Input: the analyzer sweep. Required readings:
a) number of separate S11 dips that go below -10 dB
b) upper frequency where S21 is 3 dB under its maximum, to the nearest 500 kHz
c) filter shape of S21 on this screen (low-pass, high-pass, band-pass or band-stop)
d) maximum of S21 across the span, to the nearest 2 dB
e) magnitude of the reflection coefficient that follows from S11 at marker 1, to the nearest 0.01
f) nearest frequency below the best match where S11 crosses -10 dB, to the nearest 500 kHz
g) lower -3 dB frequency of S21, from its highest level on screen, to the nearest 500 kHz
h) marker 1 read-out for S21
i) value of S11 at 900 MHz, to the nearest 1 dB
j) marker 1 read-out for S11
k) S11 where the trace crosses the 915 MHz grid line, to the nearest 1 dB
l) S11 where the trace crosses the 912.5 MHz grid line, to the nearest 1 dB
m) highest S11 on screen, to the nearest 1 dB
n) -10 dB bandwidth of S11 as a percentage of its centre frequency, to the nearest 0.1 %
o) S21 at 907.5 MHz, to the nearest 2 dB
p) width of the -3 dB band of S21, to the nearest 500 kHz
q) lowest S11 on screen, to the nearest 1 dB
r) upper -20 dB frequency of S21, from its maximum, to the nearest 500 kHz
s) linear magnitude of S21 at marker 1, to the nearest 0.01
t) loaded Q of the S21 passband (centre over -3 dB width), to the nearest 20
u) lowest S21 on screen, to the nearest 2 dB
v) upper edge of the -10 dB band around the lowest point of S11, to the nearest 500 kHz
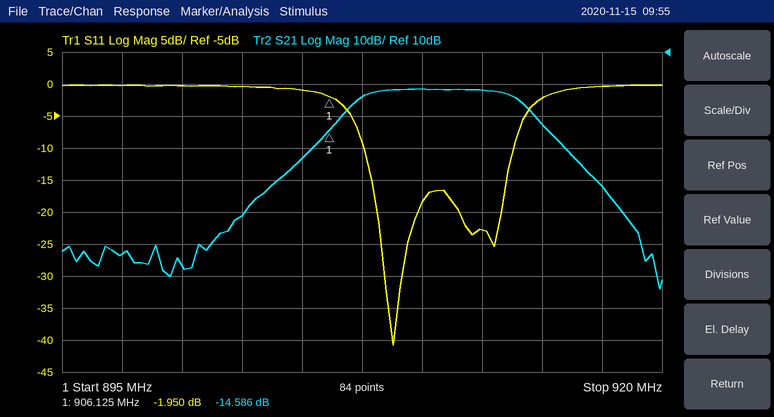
2
914.0 MHz
band-pass
-2 dB
0.80
907.5 MHz
907.5 MHz
-14.586 dB
0 dB
-1.950 dB
-2 dB
-23 dB
0 dB
0.7 %
-4 dB
6.5 MHz
-41 dB
916.0 MHz
0.19
140
-64 dB
914.0 MHz
